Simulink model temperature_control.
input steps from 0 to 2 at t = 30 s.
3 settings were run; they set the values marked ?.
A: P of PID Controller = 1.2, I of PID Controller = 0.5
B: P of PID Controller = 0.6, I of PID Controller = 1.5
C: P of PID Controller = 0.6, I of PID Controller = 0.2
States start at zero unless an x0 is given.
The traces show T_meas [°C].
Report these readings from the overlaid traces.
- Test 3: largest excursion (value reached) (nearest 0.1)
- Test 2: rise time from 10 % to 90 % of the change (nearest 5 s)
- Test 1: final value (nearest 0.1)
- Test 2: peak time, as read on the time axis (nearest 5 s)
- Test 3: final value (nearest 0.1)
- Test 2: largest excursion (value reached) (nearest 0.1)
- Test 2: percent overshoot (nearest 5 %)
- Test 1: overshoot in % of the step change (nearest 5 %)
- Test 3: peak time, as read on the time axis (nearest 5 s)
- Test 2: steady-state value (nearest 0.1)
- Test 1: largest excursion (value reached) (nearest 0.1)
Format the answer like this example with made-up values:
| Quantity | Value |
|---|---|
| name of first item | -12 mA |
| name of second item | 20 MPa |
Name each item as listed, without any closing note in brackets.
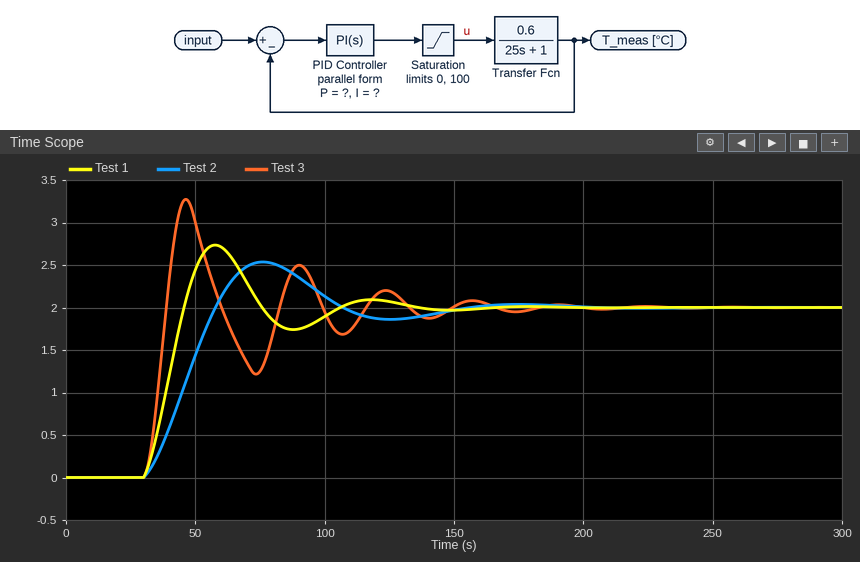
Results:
| Quantity | Value |
|---|---|
| Test 3: largest excursion (value reached) | 3.3 |
| Test 2: rise time from 10 % to 90 % of the change | 20 s |
| Test 1: final value | 2.0 |
| Test 2: peak time, as read on the time axis | 75 s |
| Test 3: final value | 2.0 |
| Test 2: largest excursion (value reached) | 2.5 |
| Test 2: percent overshoot | 25 % |
| Test 1: overshoot in % of the step change | 35 % |
| Test 3: peak time, as read on the time axis | 45 s |
| Test 2: steady-state value | 2.0 |
| Test 1: largest excursion (value reached) | 2.7 |
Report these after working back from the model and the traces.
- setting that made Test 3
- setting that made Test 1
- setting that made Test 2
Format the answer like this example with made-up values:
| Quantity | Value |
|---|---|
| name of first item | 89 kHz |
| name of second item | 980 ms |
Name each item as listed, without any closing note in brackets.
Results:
| Quantity | Value |
|---|---|
| setting that made Test 3 | B |
| setting that made Test 1 | A |
| setting that made Test 2 | C |
